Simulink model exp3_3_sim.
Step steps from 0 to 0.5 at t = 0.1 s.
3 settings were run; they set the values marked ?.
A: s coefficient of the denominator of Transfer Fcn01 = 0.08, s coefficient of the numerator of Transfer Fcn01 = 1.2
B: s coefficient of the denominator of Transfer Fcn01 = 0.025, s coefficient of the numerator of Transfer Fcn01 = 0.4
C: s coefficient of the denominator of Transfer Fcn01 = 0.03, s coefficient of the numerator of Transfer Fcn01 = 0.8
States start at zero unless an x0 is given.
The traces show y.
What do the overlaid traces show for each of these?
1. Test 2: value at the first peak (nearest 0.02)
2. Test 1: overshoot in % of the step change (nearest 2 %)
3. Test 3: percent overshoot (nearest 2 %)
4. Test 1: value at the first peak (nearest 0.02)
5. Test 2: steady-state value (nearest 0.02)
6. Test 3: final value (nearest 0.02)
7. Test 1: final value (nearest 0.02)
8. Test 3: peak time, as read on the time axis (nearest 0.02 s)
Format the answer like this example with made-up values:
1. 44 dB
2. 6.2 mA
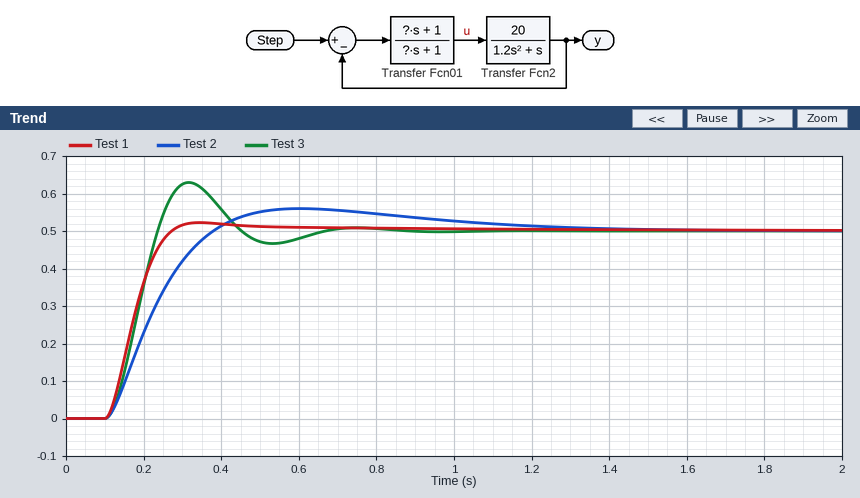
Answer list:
1. 0.56
2. 4 %
3. 26 %
4. 0.52
5. 0.50
6. 0.50
7. 0.50
8. 0.32 s
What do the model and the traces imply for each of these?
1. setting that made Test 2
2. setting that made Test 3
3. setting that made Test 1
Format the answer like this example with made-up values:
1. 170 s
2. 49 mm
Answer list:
1. B
2. A
3. C
